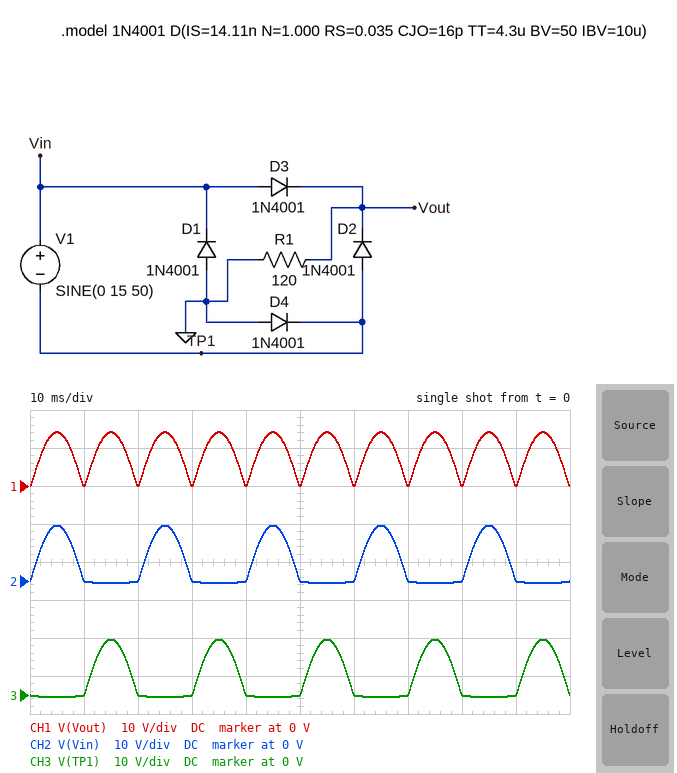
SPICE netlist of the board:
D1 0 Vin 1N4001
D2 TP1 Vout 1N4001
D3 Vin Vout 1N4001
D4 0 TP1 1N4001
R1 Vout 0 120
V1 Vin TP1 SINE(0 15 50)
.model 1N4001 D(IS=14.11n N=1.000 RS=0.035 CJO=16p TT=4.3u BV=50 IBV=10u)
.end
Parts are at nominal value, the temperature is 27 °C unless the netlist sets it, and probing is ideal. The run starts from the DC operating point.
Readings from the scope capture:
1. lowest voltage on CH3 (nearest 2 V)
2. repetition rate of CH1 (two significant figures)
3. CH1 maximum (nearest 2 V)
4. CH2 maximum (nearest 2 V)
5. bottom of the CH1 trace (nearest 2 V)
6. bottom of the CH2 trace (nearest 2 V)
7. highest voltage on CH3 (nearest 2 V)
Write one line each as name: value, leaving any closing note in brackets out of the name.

lowest voltage on CH3: 0 V
repetition rate of CH1: 100 Hz
CH1 maximum: 14 V
CH2 maximum: 14 V
bottom of the CH1 trace: 0 V
bottom of the CH2 trace: 0 V
highest voltage on CH3: 14 V
